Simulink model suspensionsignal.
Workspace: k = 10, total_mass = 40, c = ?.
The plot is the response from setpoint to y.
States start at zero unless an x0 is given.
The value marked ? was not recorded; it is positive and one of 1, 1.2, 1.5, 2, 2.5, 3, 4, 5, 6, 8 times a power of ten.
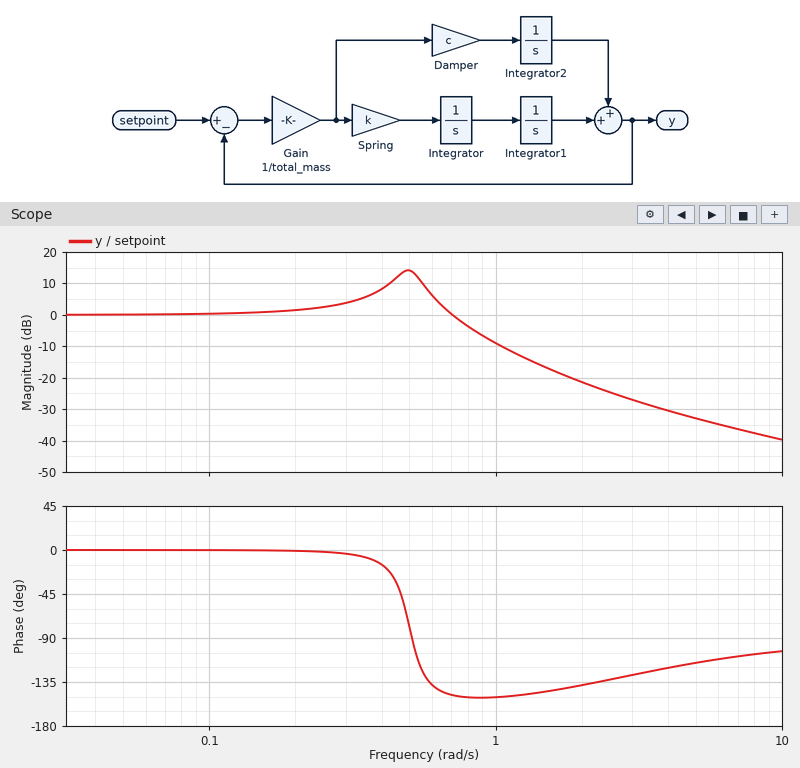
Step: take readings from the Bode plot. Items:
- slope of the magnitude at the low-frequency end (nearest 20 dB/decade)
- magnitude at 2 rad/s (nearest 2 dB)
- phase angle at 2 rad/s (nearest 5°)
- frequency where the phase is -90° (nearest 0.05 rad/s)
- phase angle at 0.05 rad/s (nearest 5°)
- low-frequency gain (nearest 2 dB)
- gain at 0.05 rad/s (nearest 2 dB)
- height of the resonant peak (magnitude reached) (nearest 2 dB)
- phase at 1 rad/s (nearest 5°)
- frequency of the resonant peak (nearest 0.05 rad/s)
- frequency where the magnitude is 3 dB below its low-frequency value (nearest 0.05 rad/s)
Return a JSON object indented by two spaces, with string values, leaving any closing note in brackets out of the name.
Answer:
{
  "slope of the magnitude at the low-frequency end": "0 dB/decade",
  "magnitude at 2 rad/s": "-22 dB",
  "phase angle at 2 rad/s": "-140°",
  "frequency where the phase is -90°": "0.50 rad/s",
  "phase angle at 0.05 rad/s": "0°",
  "low-frequency gain": "0 dB",
  "gain at 0.05 rad/s": "0 dB",
  "height of the resonant peak (magnitude reached)": "14 dB",
  "phase at 1 rad/s": "-150°",
  "frequency of the resonant peak": "0.50 rad/s",
  "frequency where the magnitude is 3 dB below its low-frequency value": "0.80 rad/s"
}
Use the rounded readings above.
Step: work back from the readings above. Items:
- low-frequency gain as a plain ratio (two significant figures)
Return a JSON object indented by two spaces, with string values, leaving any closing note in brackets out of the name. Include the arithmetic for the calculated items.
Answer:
{
  "low-frequency gain as a plain ratio": "10^(0 / 20) = 1.0"
}
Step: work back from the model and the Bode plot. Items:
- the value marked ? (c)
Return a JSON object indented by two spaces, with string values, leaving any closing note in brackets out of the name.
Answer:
{
  "the value marked ?": "4"
}
